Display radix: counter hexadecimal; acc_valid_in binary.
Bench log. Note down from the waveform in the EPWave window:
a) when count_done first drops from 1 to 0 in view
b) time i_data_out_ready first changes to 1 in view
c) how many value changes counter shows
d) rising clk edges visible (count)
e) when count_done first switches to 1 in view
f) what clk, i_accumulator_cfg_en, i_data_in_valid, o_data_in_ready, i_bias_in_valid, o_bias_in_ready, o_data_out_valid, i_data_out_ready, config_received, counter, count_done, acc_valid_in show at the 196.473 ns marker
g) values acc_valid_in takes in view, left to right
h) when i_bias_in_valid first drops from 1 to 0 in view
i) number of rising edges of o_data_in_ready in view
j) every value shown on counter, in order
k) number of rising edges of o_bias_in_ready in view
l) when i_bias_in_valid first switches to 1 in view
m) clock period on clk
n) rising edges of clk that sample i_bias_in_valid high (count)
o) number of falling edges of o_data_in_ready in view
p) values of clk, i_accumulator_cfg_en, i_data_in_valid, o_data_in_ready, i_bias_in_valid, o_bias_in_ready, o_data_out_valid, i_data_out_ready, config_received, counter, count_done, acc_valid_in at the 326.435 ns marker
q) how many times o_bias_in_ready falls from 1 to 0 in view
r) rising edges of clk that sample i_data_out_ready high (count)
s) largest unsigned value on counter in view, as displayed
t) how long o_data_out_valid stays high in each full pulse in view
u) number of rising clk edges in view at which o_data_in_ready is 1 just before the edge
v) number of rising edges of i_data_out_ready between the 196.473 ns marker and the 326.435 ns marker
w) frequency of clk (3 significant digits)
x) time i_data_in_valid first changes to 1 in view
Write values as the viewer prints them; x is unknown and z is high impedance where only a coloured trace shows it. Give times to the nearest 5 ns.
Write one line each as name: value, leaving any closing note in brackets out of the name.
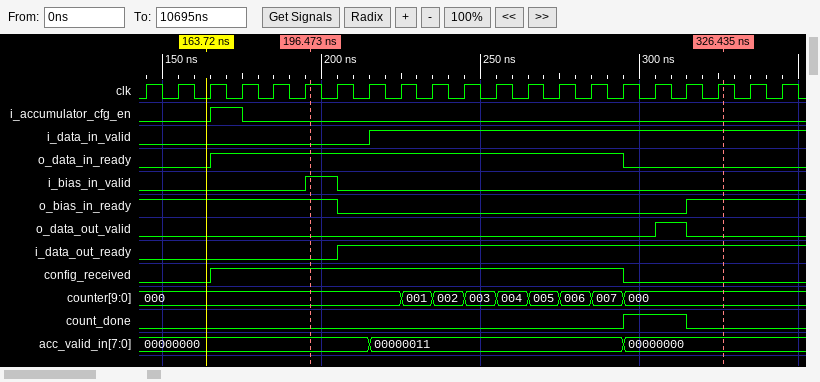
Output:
when count_done first drops from 1 to 0 in view: 315 ns
time i_data_out_ready first changes to 1 in view: 205 ns
how many value changes counter shows: 8
rising clk edges visible: 21
when count_done first switches to 1 in view: 295 ns
what clk, i_accumulator_cfg_en, i_data_in_valid, o_data_in_ready, i_bias_in_valid, o_bias_in_ready, o_data_out_valid, i_data_out_ready, config_received, counter, count_done, acc_valid_in show at the 196.473 ns marker: clk=1, i_accumulator_cfg_en=0, i_data_in_valid=0, o_data_in_ready=1, i_bias_in_valid=1, o_bias_in_ready=1, o_data_out_valid=0, i_data_out_ready=0, config_received=1, counter=000, count_done=0, acc_valid_in=00000000
values acc_valid_in takes in view, left to right: 00000000, 00000011, 00000000
when i_bias_in_valid first drops from 1 to 0 in view: 205 ns
number of rising edges of o_data_in_ready in view: 1
every value shown on counter, in order: 000, 001, 002, 003, 004, 005, 006, 007, 000
number of rising edges of o_bias_in_ready in view: 1
when i_bias_in_valid first switches to 1 in view: 195 ns
clock period on clk: 10 ns
rising edges of clk that sample i_bias_in_valid high: 1
number of falling edges of o_data_in_ready in view: 1
values of clk, i_accumulator_cfg_en, i_data_in_valid, o_data_in_ready, i_bias_in_valid, o_bias_in_ready, o_data_out_valid, i_data_out_ready, config_received, counter, count_done, acc_valid_in at the 326.435 ns marker: clk=1, i_accumulator_cfg_en=0, i_data_in_valid=1, o_data_in_ready=0, i_bias_in_valid=0, o_bias_in_ready=1, o_data_out_valid=0, i_data_out_ready=1, config_received=0, counter=000, count_done=0, acc_valid_in=00000000
how many times o_bias_in_ready falls from 1 to 0 in view: 1
rising edges of clk that sample i_data_out_ready high: 14
largest unsigned value on counter in view, as displayed: 007
how long o_data_out_valid stays high in each full pulse in view: 10 ns
number of rising clk edges in view at which o_data_in_ready is 1 just before the edge: 13
number of rising edges of i_data_out_ready between the 196.473 ns marker and the 326.435 ns marker: 1
frequency of clk: 100 MHz
time i_data_in_valid first changes to 1 in view: 215 ns
